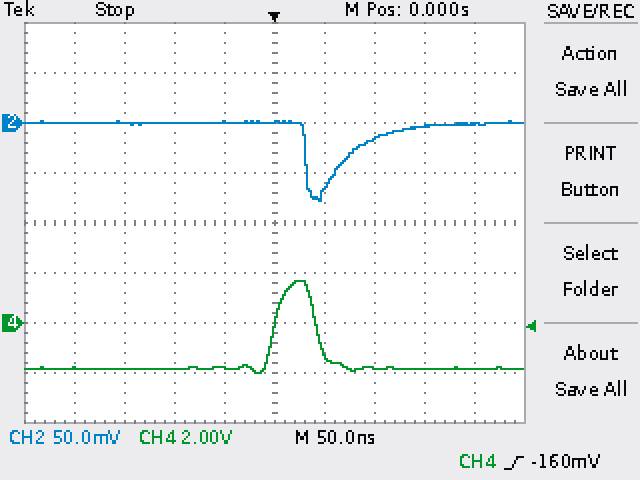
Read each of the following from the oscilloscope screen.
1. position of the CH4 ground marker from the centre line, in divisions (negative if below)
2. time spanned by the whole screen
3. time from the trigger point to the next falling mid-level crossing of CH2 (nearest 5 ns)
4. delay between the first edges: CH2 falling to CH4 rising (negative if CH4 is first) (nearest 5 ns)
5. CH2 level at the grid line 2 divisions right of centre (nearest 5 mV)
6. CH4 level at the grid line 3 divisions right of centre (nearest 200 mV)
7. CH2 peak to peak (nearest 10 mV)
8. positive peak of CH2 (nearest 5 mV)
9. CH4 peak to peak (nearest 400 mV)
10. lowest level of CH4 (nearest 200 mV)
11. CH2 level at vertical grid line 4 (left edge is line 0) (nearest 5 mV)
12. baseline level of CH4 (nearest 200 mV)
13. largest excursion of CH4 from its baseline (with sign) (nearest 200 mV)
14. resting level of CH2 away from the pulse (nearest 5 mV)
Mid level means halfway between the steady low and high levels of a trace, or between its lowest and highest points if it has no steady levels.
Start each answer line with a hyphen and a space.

- -2.0 div
- 500 ns
- 30 ns
- -30 ns
- -15 mV
- -1.8 V
- 80 mV
- 0 mV
- 3.6 V
- -2.0 V
- 0 mV
- -1.8 V
- +3.6 V
- 0 mV
